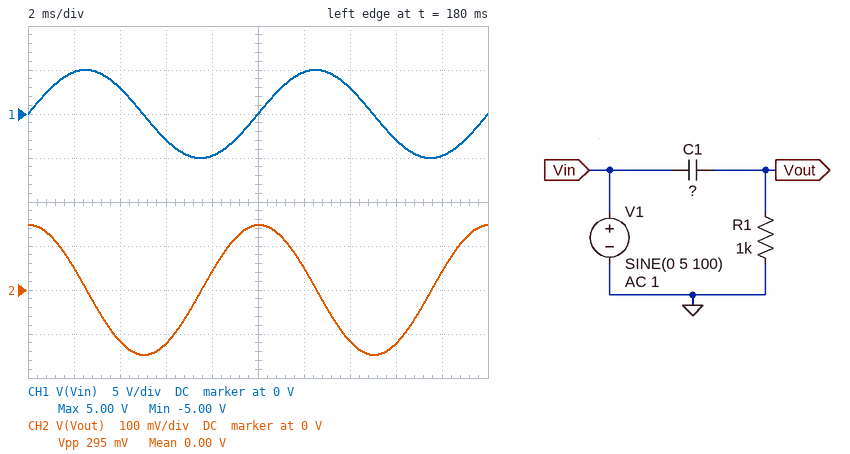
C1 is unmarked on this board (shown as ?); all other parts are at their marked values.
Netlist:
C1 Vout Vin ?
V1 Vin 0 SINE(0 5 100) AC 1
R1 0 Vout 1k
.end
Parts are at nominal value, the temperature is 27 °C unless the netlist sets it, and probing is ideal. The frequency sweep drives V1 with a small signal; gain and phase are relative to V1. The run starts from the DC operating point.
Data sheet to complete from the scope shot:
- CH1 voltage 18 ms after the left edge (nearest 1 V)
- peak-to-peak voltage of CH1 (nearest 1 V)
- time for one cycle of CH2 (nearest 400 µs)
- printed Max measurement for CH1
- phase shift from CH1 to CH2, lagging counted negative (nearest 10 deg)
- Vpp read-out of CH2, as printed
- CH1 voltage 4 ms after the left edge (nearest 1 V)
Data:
-5 V
10 V
10.0 ms
5.00 V
90 deg
295 mV
3 V
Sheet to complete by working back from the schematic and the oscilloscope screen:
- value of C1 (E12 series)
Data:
47 nF
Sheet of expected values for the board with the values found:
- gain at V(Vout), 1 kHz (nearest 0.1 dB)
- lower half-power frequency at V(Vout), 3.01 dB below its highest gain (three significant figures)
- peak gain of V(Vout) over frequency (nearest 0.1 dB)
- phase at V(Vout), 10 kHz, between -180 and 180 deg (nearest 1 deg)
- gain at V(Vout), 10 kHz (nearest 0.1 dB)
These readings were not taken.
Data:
-11.0 dB
3.39 kHz
0 dB
19 deg
-0.5 dB
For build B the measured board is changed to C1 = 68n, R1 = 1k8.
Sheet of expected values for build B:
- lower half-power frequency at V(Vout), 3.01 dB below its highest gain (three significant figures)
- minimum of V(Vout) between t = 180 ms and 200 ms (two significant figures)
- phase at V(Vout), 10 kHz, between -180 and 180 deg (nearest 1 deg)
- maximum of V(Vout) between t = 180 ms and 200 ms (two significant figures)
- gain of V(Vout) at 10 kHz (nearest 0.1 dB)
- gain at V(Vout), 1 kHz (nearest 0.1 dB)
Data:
1.30 kHz
-380 mV
7 deg
380 mV
-0.1 dB
-4.3 dB
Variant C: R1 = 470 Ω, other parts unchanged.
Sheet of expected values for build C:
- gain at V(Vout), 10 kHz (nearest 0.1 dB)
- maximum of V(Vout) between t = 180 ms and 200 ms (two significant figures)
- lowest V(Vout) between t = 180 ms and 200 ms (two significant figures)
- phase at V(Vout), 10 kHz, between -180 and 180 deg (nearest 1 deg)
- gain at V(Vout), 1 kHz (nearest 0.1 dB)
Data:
-1.8 dB
69 mV
-69 mV
36 deg
-17.2 dB
